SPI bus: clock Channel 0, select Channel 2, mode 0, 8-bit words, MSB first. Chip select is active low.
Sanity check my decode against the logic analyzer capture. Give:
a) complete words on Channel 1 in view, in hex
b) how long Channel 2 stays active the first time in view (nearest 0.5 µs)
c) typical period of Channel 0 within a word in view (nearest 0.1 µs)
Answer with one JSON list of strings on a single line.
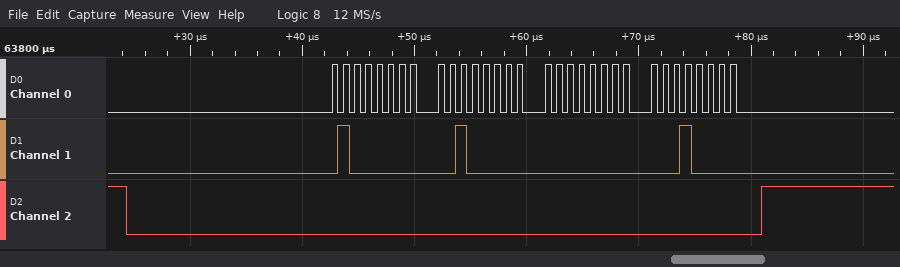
["40, 20, 00, 10", "56.5 µs", "1 µs"]
